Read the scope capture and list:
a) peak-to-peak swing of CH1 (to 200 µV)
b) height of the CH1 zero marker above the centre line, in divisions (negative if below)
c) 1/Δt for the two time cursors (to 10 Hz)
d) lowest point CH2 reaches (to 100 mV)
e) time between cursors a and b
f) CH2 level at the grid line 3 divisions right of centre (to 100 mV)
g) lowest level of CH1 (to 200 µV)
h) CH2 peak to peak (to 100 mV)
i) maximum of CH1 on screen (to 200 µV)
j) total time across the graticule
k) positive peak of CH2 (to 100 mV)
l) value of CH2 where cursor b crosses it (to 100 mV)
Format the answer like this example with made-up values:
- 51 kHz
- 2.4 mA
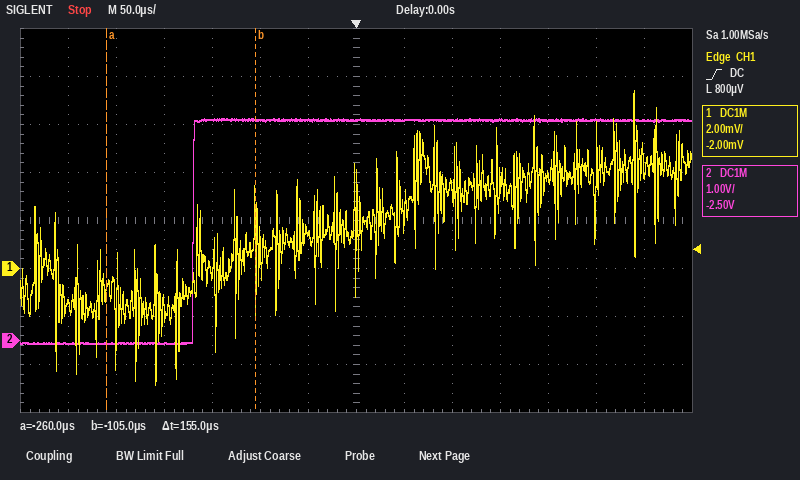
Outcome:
- 12.2 mV
- -1.0 div
- 6.45 kHz
- -100 mV
- 155 µs
- 4.6 V
- -4.8 mV
- 4.7 V
- 7.4 mV
- 700 µs
- 4.6 V
- 4.6 V
